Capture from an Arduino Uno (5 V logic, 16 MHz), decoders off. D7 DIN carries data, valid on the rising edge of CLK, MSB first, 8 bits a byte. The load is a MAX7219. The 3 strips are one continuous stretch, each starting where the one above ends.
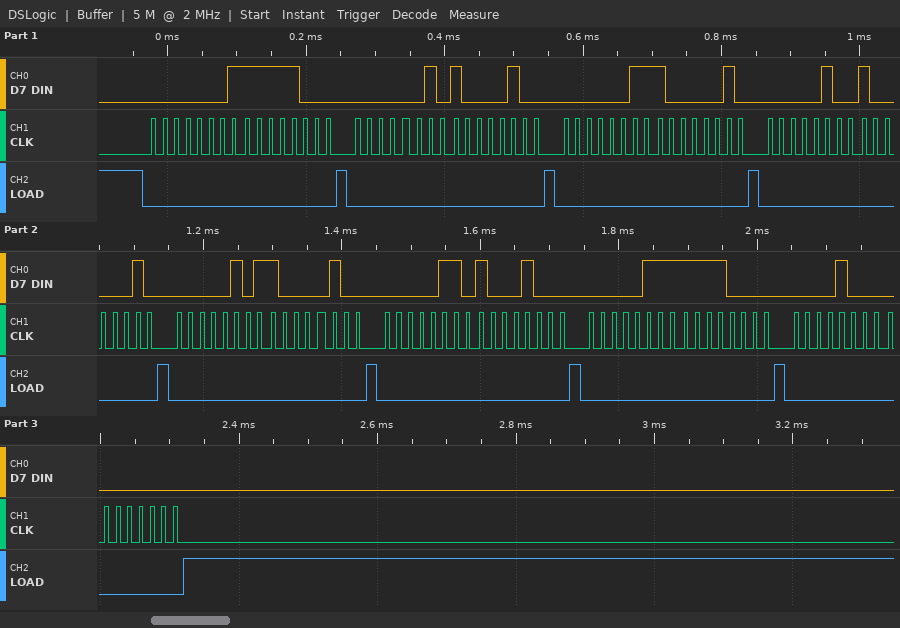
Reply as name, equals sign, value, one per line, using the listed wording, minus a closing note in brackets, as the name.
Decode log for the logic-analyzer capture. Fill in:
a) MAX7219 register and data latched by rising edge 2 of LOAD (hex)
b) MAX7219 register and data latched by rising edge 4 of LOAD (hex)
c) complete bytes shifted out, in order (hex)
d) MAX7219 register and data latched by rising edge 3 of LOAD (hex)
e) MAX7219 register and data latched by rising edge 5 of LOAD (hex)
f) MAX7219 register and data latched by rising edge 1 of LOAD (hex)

MAX7219 register and data latched by rising edge 2 of LOAD = register 0x2, data 0x84
MAX7219 register and data latched by rising edge 4 of LOAD = register 0x4, data 0x82
complete bytes shifted out, in order = 01 F8 02 84 03 82 04 82 05 84 06 88 07 F0 08 00
MAX7219 register and data latched by rising edge 3 of LOAD = register 0x3, data 0x82
MAX7219 register and data latched by rising edge 5 of LOAD = register 0x5, data 0x84
MAX7219 register and data latched by rising edge 1 of LOAD = register 0x1, data 0xF8
